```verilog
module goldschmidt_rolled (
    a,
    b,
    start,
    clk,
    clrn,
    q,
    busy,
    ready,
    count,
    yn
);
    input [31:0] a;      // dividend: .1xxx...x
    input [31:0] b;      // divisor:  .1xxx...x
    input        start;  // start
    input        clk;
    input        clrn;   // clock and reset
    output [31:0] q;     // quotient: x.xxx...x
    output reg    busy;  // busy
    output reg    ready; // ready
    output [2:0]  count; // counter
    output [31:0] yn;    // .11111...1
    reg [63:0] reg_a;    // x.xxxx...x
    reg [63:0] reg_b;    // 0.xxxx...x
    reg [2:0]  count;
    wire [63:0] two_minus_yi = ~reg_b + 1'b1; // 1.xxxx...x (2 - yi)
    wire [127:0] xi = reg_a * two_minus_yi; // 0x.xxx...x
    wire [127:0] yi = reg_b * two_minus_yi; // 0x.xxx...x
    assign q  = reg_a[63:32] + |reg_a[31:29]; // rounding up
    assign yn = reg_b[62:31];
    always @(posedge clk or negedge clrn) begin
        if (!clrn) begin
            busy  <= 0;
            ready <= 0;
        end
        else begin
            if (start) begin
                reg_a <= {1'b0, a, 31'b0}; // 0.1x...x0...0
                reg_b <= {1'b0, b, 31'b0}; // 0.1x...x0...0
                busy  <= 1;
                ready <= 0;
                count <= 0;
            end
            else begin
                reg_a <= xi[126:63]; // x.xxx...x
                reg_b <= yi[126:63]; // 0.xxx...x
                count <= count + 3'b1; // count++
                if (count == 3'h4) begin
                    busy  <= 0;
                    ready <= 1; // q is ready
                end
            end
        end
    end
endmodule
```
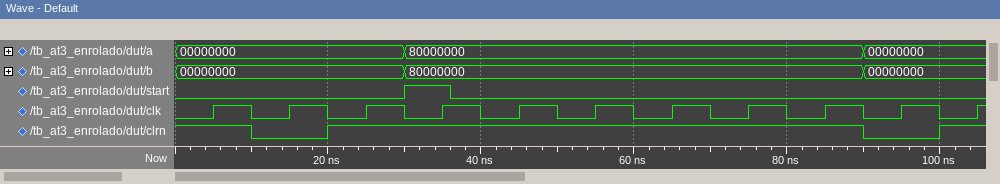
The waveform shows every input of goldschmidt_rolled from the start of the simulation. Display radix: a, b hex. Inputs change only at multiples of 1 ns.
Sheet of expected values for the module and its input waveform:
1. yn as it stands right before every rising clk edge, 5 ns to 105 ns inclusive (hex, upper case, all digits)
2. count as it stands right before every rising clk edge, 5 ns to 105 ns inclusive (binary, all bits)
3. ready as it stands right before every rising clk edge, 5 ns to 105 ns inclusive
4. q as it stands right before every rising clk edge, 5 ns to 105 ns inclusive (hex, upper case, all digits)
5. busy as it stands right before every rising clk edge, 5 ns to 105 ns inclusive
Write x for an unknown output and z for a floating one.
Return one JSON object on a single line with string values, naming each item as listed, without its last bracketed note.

{"yn as it stands right before every rising clk edge, 5 ns to 105 ns inclusive": "x, x, x, x, 80000000, C0000000, F0000000, FF000000, FFFF0000, FFFFFFFF, FFFFFFFF", "count as it stands right before every rising clk edge, 5 ns to 105 ns inclusive": "x, x, x, x, 000, 001, 010, 011, 100, 101, 101", "ready as it stands right before every rising clk edge, 5 ns to 105 ns inclusive": "x 0 0 0 0 0 0 0 0 0 0", "q as it stands right before every rising clk edge, 5 ns to 105 ns inclusive": "x, x, x, x, 40000000, 60000000, 78000000, 7F800000, 7FFF8000, 80000000, 80000000", "busy as it stands right before every rising clk edge, 5 ns to 105 ns inclusive": "x 0 0 0 1 1 1 1 1 0 0"}
